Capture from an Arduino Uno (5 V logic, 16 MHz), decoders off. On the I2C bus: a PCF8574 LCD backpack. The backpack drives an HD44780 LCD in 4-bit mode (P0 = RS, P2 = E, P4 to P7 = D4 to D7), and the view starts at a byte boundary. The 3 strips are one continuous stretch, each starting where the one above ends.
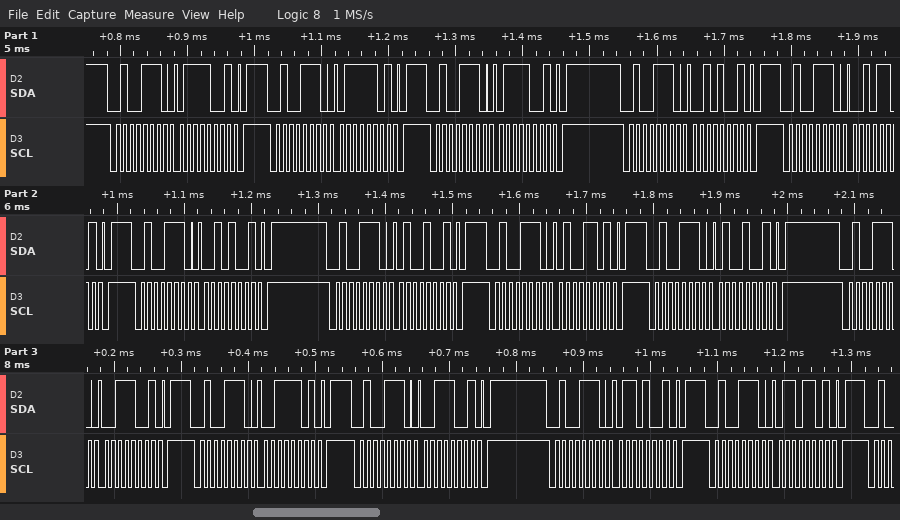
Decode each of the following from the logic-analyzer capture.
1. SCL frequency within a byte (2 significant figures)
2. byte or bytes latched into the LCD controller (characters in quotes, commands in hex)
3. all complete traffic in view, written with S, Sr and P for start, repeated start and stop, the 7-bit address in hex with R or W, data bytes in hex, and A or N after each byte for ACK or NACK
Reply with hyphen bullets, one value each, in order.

- 100 kHz
- 'r' 'C'
- S 27W A 79 A P S 27W A 7D A P S 27W A 79 A P S 27W A 29 A P S 27W A 2D A P S 27W A 29 A P S 27W A 49 A P S 27W A 4D A P S 27W A 49 A P S 27W A 39 A P S 27W A 3D A P S 27W A 39 A P S 27W A 69 A P S 27W A 6D A P
